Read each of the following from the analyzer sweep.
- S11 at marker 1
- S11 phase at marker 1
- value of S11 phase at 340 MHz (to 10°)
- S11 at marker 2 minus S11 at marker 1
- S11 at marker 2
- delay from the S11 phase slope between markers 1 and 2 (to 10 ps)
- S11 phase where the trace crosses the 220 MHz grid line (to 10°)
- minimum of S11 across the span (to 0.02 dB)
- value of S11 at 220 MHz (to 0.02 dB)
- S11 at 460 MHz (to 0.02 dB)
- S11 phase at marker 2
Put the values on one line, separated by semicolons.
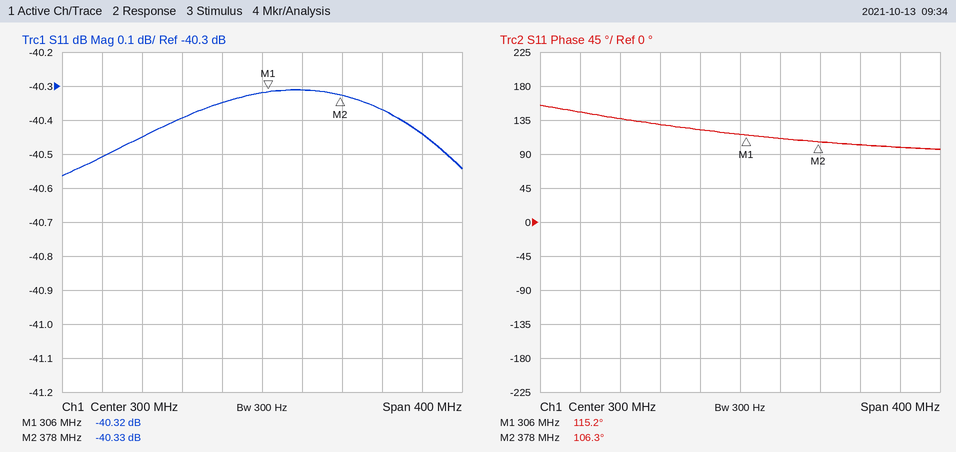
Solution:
-40.32 dB; 115.2°; 110°; -0.01 dB; -40.33 dB; 340 ps; 130°; -40.56 dB; -40.40 dB; -40.44 dB; 106.3°
